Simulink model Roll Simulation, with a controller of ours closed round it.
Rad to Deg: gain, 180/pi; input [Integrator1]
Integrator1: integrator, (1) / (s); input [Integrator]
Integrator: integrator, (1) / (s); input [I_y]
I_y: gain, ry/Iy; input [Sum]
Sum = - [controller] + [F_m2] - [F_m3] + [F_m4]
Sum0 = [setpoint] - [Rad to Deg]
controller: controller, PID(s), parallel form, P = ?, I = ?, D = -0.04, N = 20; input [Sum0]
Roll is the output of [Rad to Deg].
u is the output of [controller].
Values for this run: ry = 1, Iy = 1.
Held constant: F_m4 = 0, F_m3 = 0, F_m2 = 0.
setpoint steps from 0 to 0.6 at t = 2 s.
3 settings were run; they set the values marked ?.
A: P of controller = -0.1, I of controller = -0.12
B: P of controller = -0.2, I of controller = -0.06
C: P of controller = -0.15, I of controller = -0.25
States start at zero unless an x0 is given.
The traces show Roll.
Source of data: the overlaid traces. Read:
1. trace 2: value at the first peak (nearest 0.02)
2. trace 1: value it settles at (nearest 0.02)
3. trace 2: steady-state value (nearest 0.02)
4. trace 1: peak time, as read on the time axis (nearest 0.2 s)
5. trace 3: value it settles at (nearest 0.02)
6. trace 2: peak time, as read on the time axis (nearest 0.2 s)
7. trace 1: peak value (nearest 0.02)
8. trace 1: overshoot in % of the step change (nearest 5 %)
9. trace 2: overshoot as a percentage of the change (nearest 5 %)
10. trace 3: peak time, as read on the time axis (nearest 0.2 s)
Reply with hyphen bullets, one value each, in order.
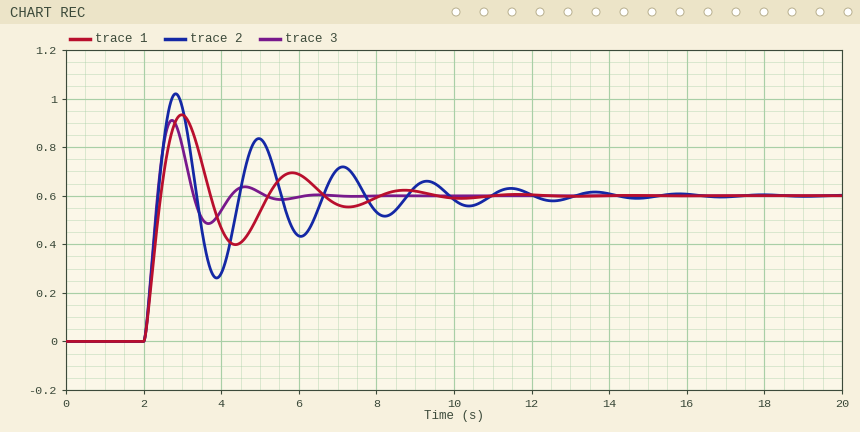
- 1.02
- 0.60
- 0.60
- 3.0 s
- 0.60
- 2.8 s
- 0.94
- 55 %
- 70 %
- 2.8 s
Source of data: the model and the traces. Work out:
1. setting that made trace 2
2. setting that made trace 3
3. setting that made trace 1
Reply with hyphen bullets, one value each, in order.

- C
- B
- A
